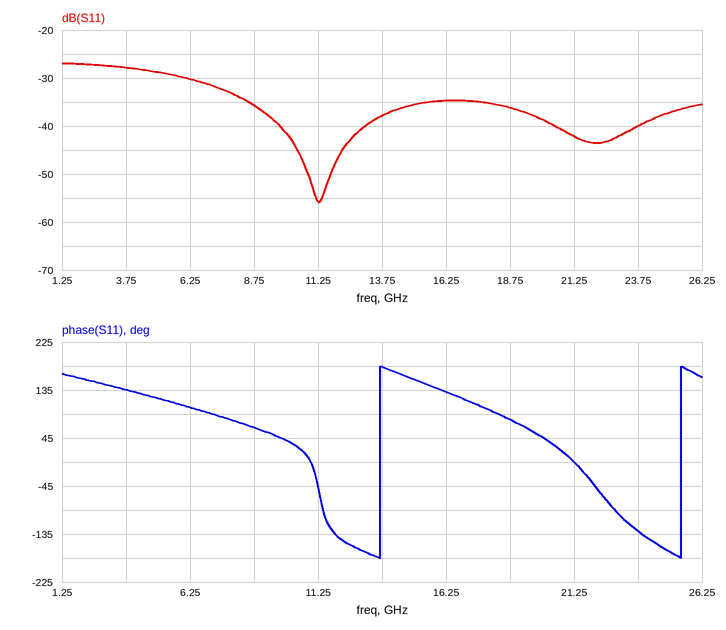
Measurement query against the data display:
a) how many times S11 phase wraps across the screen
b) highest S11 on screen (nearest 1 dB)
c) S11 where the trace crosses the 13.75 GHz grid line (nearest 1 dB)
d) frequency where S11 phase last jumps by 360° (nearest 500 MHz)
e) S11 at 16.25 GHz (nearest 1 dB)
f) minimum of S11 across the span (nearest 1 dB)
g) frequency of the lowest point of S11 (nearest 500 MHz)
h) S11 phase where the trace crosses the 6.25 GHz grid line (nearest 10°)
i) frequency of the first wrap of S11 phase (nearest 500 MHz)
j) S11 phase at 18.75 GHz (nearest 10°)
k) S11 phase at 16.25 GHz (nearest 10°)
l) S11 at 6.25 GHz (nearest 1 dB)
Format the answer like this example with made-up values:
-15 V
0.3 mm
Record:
2
-27 dB
-38 dB
25.5 GHz
-35 dB
-56 dB
11.5 GHz
100°
13.5 GHz
80°
130°
-30 dB
